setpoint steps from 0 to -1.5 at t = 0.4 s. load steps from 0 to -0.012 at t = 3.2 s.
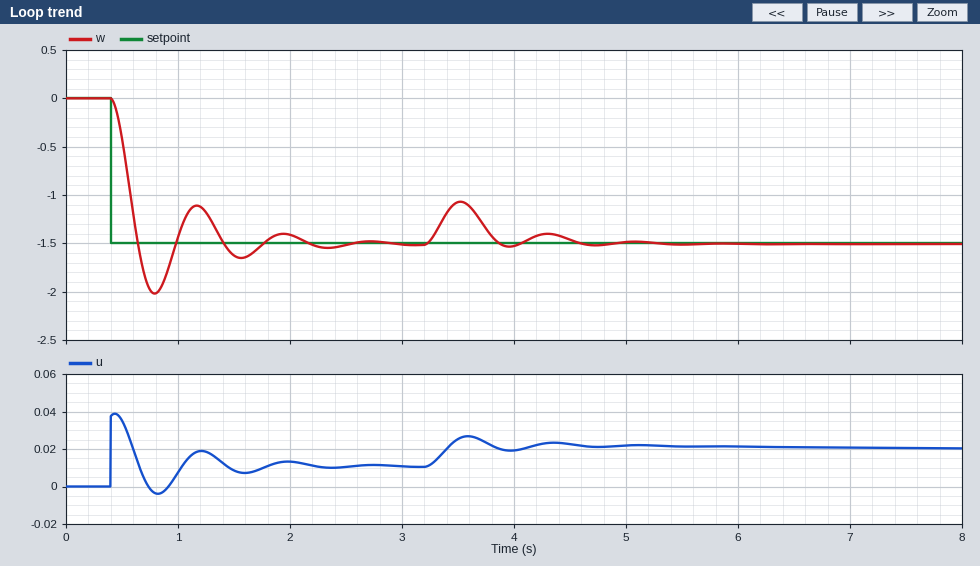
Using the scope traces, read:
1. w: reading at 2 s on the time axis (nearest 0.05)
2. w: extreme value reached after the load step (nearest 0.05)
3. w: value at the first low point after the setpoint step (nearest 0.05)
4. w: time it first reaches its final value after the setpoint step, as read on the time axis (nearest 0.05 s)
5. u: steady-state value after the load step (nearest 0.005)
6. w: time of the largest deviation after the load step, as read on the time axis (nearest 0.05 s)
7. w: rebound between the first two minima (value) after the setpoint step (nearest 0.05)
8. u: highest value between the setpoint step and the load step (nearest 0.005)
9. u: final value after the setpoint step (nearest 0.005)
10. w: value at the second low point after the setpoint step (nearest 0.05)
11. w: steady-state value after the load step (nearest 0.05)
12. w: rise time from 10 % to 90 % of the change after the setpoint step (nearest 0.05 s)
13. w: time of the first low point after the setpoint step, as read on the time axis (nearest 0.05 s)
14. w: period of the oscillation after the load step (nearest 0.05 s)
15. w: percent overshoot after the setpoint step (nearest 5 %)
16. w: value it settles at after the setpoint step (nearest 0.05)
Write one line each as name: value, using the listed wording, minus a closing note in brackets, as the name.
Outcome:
w: reading at 2 s on the time axis: -1.40
w: extreme value reached after the load step: -1.05
w: value at the first low point after the setpoint step: -2.00
w: time it first reaches its final value after the setpoint step, as read on the time axis: 0.65 s
u: steady-state value after the load step: 0.020
w: time of the largest deviation after the load step, as read on the time axis: 3.50 s
w: rebound between the first two minima (value) after the setpoint step: -1.10
u: highest value between the setpoint step and the load step: 0.040
u: final value after the setpoint step: 0.010
w: value at the second low point after the setpoint step: -1.65
w: steady-state value after the load step: -1.50
w: rise time from 10 % to 90 % of the change after the setpoint step: 0.15 s
w: time of the first low point after the setpoint step, as read on the time axis: 0.80 s
w: period of the oscillation after the load step: 0.80 s
w: percent overshoot after the setpoint step: 35 %
w: value it settles at after the setpoint step: -1.50
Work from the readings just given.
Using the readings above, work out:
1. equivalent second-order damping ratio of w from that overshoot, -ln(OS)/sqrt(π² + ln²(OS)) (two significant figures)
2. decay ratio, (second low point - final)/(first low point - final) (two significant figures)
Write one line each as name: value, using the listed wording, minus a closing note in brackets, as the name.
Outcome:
equivalent second-order damping ratio of w from that overshoot, -ln(OS)/sqrt(π² + ln²(OS)): 0.32
decay ratio, (second low point - final)/(first low point - final): 0.30
